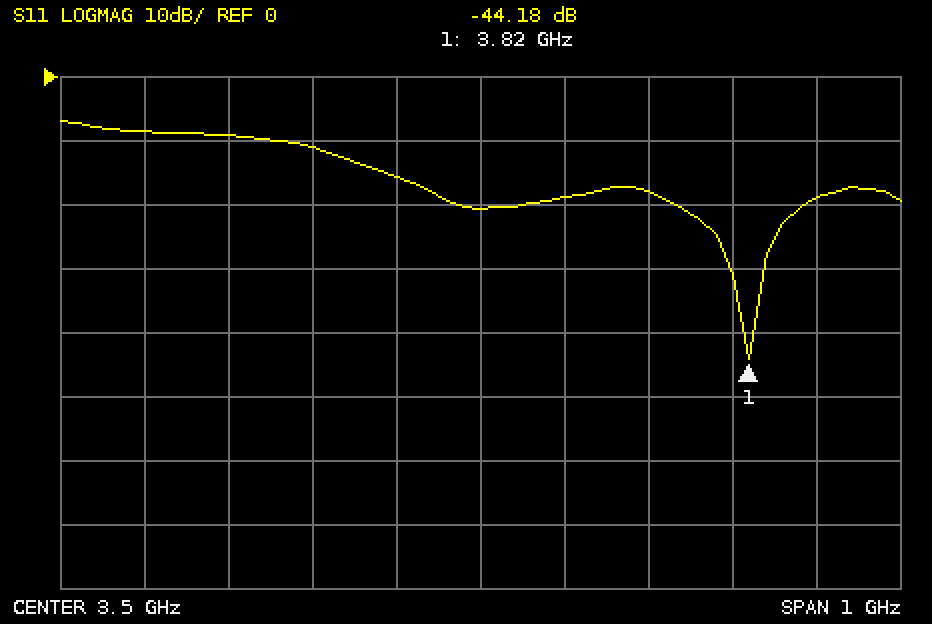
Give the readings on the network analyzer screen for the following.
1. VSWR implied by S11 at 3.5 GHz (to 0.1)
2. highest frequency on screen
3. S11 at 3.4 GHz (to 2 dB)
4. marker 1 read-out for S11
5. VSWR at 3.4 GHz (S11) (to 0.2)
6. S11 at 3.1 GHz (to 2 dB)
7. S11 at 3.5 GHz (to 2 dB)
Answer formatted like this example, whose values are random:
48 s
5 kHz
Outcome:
1.2
4 GHz
-16 dB
-44.18 dB
1.4
-8 dB
-20 dB
